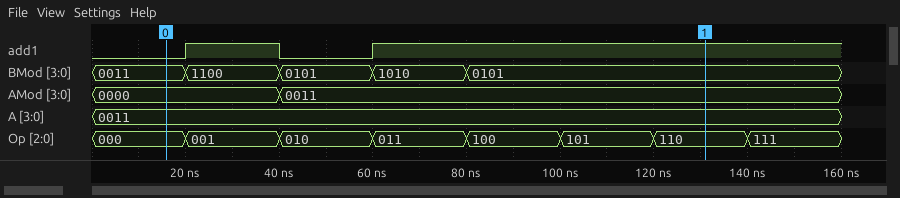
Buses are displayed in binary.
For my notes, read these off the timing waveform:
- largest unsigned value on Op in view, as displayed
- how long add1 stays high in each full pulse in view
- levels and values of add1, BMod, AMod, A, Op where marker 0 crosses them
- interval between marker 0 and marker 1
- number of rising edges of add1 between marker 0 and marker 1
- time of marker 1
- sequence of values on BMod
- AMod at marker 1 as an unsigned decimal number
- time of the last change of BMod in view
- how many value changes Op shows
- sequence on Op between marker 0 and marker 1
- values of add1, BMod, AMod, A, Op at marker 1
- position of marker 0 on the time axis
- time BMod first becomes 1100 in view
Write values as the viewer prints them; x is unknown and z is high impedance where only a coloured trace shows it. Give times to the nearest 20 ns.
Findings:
111
20 ns
add1=0, BMod=0011, AMod=0000, A=0011, Op=000
120 ns
2
140 ns
0011, 1100, 0101, 1010, 0101
3
80 ns
7
000, 001, 010, 011, 100, 101, 110
add1=1, BMod=0101, AMod=0011, A=0011, Op=110
20 ns
20 ns
